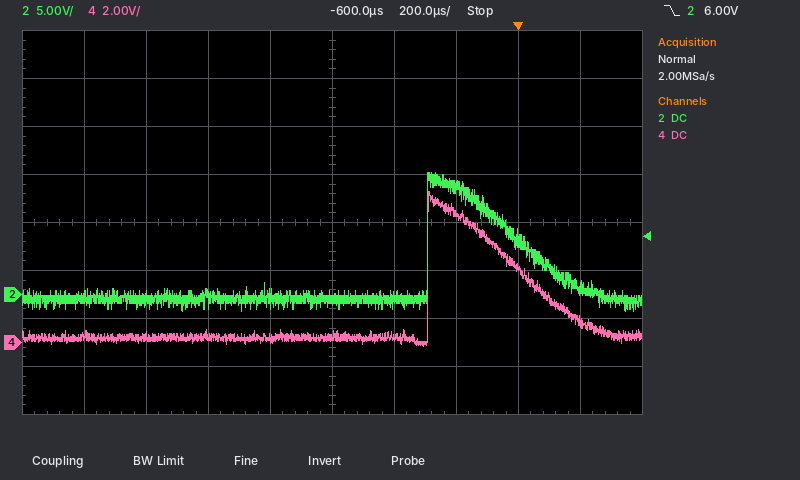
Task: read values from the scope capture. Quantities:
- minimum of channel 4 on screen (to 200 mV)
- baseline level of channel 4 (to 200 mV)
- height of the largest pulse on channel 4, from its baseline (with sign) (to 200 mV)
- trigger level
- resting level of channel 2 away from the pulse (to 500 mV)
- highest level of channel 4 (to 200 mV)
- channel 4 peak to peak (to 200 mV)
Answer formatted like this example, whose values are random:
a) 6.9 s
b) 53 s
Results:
a) -200 mV
b) 200 mV
c) +6.0 V
d) 6.00 V
e) -500 mV
f) 6.2 V
g) 6.4 V
